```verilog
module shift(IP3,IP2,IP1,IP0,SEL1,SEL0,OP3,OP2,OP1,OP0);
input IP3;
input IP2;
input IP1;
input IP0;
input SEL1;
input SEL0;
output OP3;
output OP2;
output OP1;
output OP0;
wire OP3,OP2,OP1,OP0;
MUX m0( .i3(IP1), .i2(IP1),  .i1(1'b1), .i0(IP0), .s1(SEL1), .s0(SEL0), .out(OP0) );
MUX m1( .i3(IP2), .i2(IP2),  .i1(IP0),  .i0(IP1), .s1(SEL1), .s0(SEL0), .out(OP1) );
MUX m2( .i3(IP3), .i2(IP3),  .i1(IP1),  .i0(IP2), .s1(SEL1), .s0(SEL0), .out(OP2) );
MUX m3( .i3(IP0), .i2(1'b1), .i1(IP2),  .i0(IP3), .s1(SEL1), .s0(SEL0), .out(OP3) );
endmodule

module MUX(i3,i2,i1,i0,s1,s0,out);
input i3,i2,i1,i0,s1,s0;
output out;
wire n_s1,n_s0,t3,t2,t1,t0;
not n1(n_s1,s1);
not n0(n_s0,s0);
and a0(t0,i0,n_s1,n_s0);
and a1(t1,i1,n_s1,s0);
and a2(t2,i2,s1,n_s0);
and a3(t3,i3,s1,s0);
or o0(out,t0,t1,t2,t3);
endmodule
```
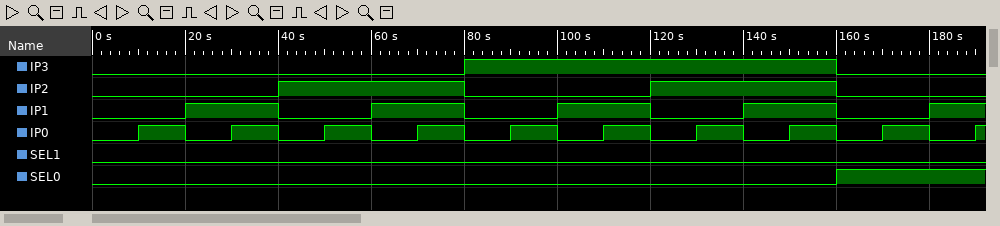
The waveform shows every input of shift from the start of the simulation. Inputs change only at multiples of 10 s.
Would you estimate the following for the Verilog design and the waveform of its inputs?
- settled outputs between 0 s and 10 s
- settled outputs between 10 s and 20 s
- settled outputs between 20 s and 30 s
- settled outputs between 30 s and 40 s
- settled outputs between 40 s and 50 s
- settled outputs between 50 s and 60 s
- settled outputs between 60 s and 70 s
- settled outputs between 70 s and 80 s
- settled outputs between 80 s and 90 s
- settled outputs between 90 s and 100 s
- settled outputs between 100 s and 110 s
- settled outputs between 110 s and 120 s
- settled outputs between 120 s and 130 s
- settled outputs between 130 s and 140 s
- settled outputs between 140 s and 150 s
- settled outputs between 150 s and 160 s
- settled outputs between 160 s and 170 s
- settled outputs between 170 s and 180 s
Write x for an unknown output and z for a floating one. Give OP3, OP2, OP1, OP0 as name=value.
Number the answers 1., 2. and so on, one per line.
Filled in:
1. OP3=0, OP2=0, OP1=0, OP0=0
2. OP3=0, OP2=0, OP1=0, OP0=1
3. OP3=0, OP2=0, OP1=1, OP0=0
4. OP3=0, OP2=0, OP1=1, OP0=1
5. OP3=0, OP2=1, OP1=0, OP0=0
6. OP3=0, OP2=1, OP1=0, OP0=1
7. OP3=0, OP2=1, OP1=1, OP0=0
8. OP3=0, OP2=1, OP1=1, OP0=1
9. OP3=1, OP2=0, OP1=0, OP0=0
10. OP3=1, OP2=0, OP1=0, OP0=1
11. OP3=1, OP2=0, OP1=1, OP0=0
12. OP3=1, OP2=0, OP1=1, OP0=1
13. OP3=1, OP2=1, OP1=0, OP0=0
14. OP3=1, OP2=1, OP1=0, OP0=1
15. OP3=1, OP2=1, OP1=1, OP0=0
16. OP3=1, OP2=1, OP1=1, OP0=1
17. OP3=0, OP2=0, OP1=0, OP0=1
18. OP3=0, OP2=0, OP1=1, OP0=1
